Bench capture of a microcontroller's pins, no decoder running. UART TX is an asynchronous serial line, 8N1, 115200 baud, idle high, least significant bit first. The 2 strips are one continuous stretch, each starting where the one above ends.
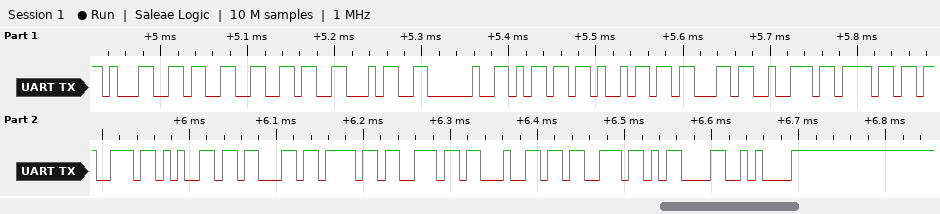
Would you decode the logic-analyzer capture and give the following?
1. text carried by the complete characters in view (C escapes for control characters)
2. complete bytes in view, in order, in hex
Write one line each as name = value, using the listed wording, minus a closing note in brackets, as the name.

text carried by the complete characters in view = "1364 microseconds\r\n"
complete bytes in view, in order, in hex = 31 33 36 34 20 6D 69 63 72 6F 73 65 63 6F 6E 64 73 0D 0A
